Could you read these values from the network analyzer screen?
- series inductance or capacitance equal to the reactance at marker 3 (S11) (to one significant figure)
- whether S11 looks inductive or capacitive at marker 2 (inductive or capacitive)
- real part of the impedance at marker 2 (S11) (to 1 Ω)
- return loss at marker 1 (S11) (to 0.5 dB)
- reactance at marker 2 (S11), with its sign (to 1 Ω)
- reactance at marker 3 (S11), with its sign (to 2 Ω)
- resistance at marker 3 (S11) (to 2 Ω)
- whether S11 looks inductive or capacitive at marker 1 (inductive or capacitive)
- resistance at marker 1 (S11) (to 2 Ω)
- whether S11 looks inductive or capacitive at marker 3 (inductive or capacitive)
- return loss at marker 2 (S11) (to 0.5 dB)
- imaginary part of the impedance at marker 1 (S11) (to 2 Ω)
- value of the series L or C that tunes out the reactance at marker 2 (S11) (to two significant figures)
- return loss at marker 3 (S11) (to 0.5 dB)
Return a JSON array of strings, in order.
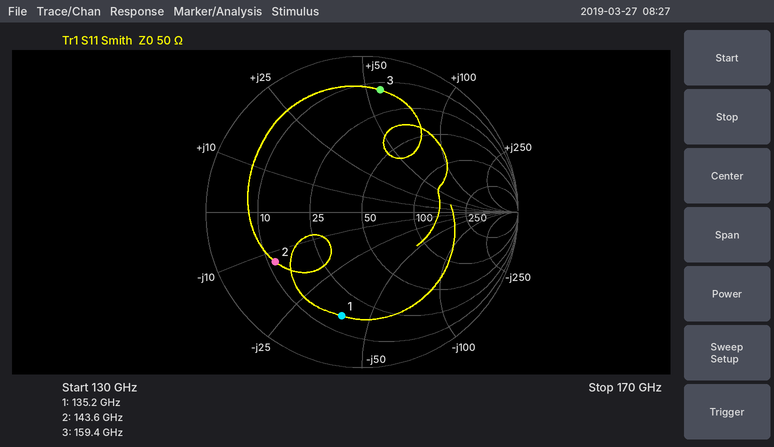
["60 pH", "capacitive", "12 Ω", "3.5 dB", "-13 Ω", "+56 Ω", "14 Ω", "capacitive", "16 Ω", "inductive", "4.0 dB", "-38 Ω", "14 pH", "2.0 dB"]
